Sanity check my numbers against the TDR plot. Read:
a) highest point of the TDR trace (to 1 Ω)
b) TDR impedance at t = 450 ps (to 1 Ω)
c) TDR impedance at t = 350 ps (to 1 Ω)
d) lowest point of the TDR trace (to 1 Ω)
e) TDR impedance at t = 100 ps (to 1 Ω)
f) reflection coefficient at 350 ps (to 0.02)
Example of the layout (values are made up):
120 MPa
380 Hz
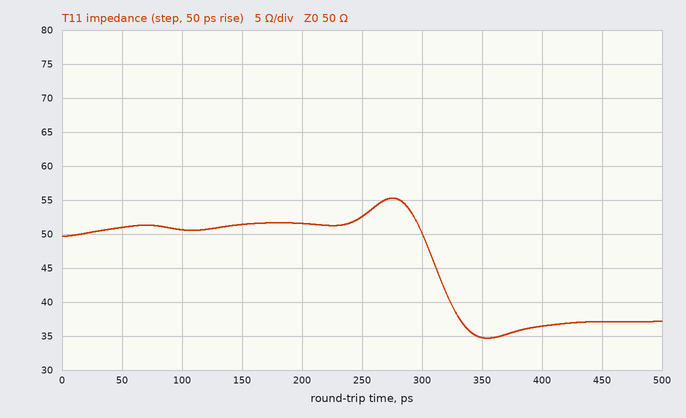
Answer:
55 Ω
37 Ω
35 Ω
35 Ω
51 Ω
-0.18
